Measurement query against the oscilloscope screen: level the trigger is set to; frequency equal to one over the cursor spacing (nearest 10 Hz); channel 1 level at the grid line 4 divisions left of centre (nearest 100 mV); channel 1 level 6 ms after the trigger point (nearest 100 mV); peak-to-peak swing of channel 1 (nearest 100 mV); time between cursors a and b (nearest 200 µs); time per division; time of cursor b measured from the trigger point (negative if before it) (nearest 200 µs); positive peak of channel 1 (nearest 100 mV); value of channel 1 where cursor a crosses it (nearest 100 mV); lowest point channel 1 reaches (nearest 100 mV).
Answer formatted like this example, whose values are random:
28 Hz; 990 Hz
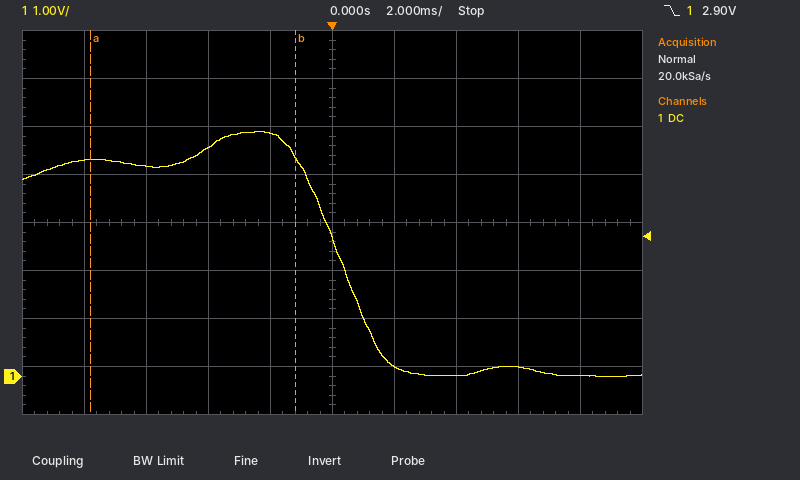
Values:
2.90 V; 150 Hz; 4.5 V; 200 mV; 5.1 V; 6.6 ms; 2 ms; -1.2 ms; 5.1 V; 4.5 V; 0.0 V
